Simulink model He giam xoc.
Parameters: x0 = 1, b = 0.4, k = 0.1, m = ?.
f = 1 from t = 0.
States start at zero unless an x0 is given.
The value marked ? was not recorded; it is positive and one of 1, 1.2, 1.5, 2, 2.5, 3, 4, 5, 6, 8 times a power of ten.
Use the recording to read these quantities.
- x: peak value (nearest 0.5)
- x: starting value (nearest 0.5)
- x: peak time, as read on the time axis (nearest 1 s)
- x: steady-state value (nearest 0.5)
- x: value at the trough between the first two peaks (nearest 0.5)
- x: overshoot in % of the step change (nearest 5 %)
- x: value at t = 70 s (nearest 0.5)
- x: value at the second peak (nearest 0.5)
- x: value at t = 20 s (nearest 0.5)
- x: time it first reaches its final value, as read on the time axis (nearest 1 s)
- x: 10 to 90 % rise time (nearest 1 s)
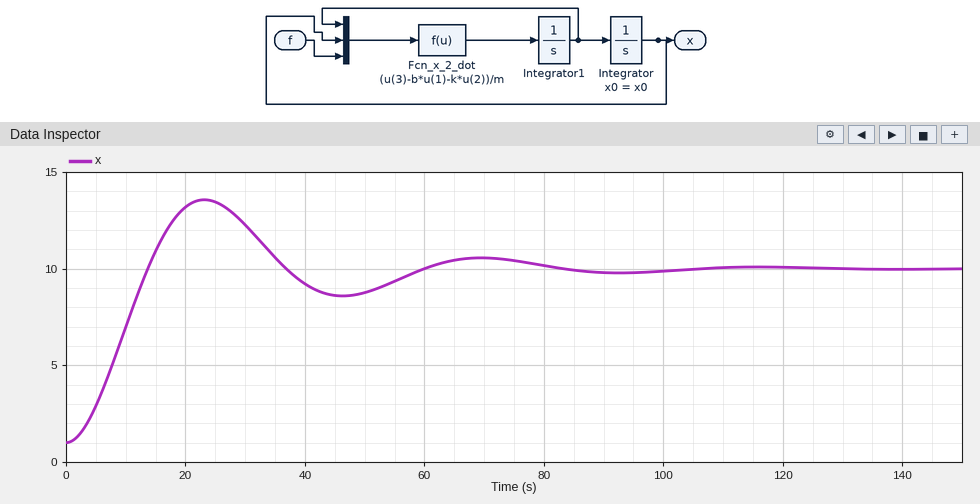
13.5
1.0
23 s
10.0
8.5
40 %
10.5
10.5
13.0
14 s
9 s
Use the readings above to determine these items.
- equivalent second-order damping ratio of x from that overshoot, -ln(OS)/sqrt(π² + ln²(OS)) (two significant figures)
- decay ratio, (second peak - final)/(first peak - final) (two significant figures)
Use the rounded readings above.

0.28
0.14
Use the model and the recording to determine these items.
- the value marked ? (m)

5
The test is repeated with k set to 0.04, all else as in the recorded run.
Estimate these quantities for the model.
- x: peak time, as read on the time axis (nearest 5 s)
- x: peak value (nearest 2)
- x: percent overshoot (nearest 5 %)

40 s
30
20 %
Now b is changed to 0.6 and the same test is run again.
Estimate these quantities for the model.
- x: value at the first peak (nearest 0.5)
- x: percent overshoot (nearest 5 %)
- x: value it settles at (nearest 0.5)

12.0
25 %
10.0
